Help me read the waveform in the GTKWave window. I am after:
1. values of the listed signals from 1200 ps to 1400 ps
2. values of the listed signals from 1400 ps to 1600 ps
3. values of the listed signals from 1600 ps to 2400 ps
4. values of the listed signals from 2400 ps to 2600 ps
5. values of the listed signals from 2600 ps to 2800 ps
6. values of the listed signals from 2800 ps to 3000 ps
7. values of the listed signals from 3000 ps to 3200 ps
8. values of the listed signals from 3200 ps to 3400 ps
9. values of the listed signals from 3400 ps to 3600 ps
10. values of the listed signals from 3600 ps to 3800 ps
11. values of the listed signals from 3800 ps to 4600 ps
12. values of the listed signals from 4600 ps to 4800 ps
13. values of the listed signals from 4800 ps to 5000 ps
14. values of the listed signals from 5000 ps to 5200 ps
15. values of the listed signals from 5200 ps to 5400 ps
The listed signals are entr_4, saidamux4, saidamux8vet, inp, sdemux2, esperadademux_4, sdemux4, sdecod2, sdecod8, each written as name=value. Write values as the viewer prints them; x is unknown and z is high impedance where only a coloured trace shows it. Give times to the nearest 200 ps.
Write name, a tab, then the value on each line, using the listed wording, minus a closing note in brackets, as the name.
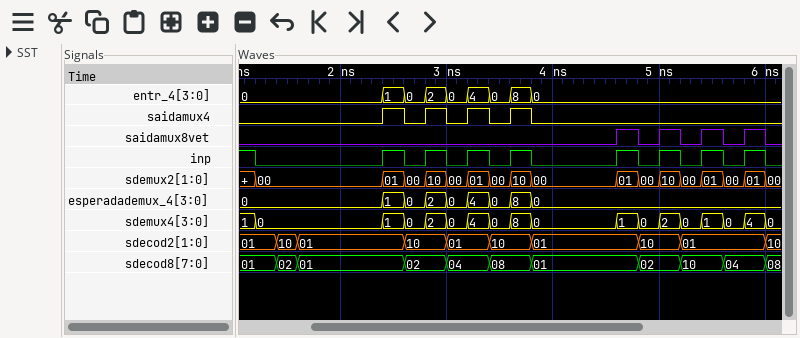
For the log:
values of the listed signals from 1200 ps to 1400 ps	entr_4=0, saidamux4=0, saidamux8vet=0, inp=0, sdemux2=00, esperadademux_4=0, sdemux4=0, sdecod2=01, sdecod8=01
values of the listed signals from 1400 ps to 1600 ps	entr_4=0, saidamux4=0, saidamux8vet=0, inp=0, sdemux2=00, esperadademux_4=0, sdemux4=0, sdecod2=10, sdecod8=02
values of the listed signals from 1600 ps to 2400 ps	entr_4=0, saidamux4=0, saidamux8vet=0, inp=0, sdemux2=00, esperadademux_4=0, sdemux4=0, sdecod2=01, sdecod8=01
values of the listed signals from 2400 ps to 2600 ps	entr_4=1, saidamux4=1, saidamux8vet=0, inp=1, sdemux2=01, esperadademux_4=1, sdemux4=1, sdecod2=01, sdecod8=01
values of the listed signals from 2600 ps to 2800 ps	entr_4=0, saidamux4=0, saidamux8vet=0, inp=0, sdemux2=00, esperadademux_4=0, sdemux4=0, sdecod2=10, sdecod8=02
values of the listed signals from 2800 ps to 3000 ps	entr_4=2, saidamux4=1, saidamux8vet=0, inp=1, sdemux2=10, esperadademux_4=2, sdemux4=2, sdecod2=10, sdecod8=02
values of the listed signals from 3000 ps to 3200 ps	entr_4=0, saidamux4=0, saidamux8vet=0, inp=0, sdemux2=00, esperadademux_4=0, sdemux4=0, sdecod2=01, sdecod8=04
values of the listed signals from 3200 ps to 3400 ps	entr_4=4, saidamux4=1, saidamux8vet=0, inp=1, sdemux2=01, esperadademux_4=4, sdemux4=4, sdecod2=01, sdecod8=04
values of the listed signals from 3400 ps to 3600 ps	entr_4=0, saidamux4=0, saidamux8vet=0, inp=0, sdemux2=00, esperadademux_4=0, sdemux4=0, sdecod2=10, sdecod8=08
values of the listed signals from 3600 ps to 3800 ps	entr_4=8, saidamux4=1, saidamux8vet=0, inp=1, sdemux2=10, esperadademux_4=8, sdemux4=8, sdecod2=10, sdecod8=08
values of the listed signals from 3800 ps to 4600 ps	entr_4=0, saidamux4=0, saidamux8vet=0, inp=0, sdemux2=00, esperadademux_4=0, sdemux4=0, sdecod2=01, sdecod8=01
values of the listed signals from 4600 ps to 4800 ps	entr_4=0, saidamux4=0, saidamux8vet=1, inp=1, sdemux2=01, esperadademux_4=0, sdemux4=1, sdecod2=01, sdecod8=01
values of the listed signals from 4800 ps to 5000 ps	entr_4=0, saidamux4=0, saidamux8vet=0, inp=0, sdemux2=00, esperadademux_4=0, sdemux4=0, sdecod2=10, sdecod8=02
values of the listed signals from 5000 ps to 5200 ps	entr_4=0, saidamux4=0, saidamux8vet=1, inp=1, sdemux2=10, esperadademux_4=0, sdemux4=2, sdecod2=10, sdecod8=02
values of the listed signals from 5200 ps to 5400 ps	entr_4=0, saidamux4=0, saidamux8vet=0, inp=0, sdemux2=00, esperadademux_4=0, sdemux4=0, sdecod2=01, sdecod8=10
